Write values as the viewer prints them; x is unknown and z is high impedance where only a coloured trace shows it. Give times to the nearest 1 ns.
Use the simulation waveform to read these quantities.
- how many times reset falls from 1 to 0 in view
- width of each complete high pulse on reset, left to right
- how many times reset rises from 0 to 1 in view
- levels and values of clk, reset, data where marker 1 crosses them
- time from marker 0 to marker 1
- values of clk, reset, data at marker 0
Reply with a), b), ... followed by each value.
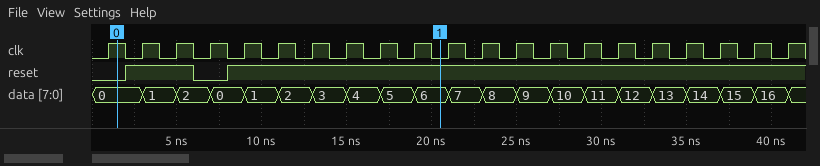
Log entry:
a) 1
b) 4 ns
c) 2
d) clk=0, reset=1, data=6
e) 19 ns
f) clk=1, reset=0, data=0
